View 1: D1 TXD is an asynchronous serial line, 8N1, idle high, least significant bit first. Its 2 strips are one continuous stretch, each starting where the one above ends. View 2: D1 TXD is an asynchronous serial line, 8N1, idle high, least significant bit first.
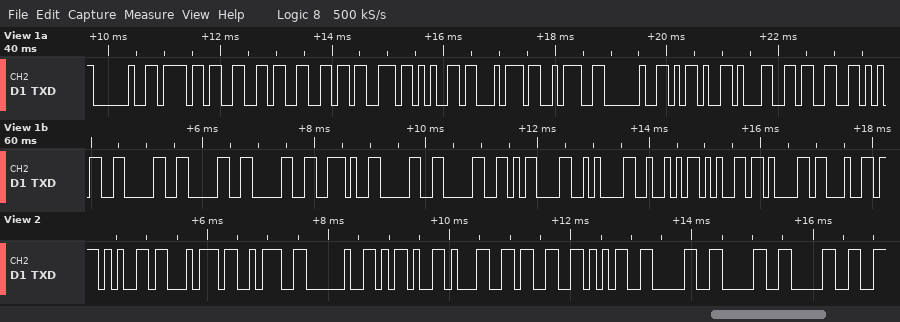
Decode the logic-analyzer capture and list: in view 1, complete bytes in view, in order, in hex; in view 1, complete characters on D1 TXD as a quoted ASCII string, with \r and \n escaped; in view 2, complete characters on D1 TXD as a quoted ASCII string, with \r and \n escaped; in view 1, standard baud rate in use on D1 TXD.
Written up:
20 6F 66 66 73 65 74 3A 20 2D 31 33 35 30 30 30 2E 30 30 0D 0A 52 65 61 64
" offset: -135000.00\r\nRead"
"et: -135000"
9600 baud
